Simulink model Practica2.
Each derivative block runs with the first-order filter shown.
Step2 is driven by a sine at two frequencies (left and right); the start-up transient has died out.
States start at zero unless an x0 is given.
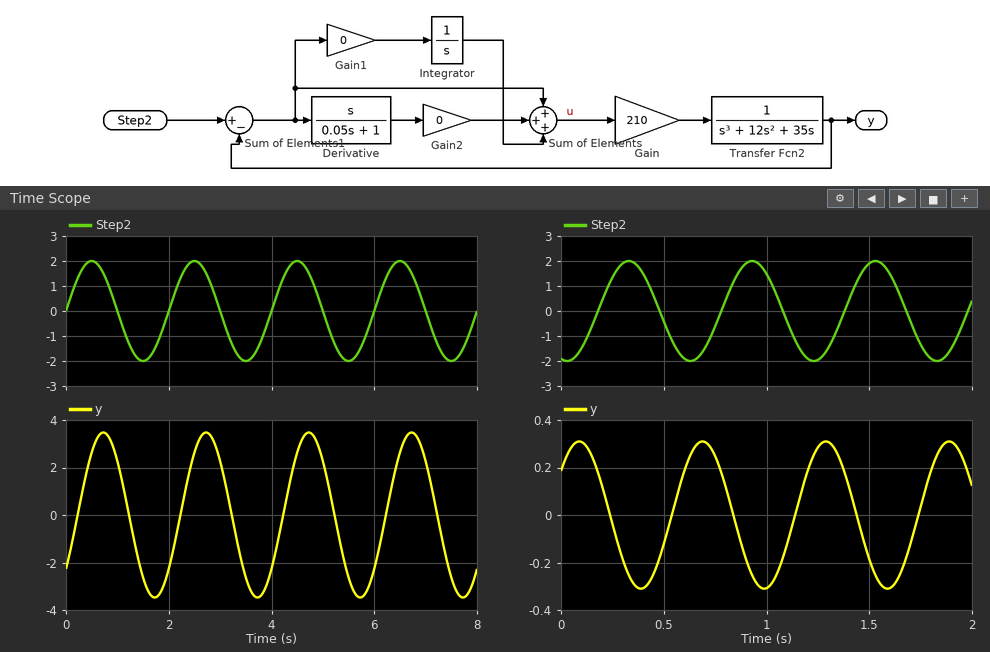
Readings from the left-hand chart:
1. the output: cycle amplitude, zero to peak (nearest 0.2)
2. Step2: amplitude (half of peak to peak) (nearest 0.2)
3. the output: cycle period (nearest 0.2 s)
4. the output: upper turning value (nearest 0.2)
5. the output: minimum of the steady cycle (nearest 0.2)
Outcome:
3.4
2.0
2.0 s
3.4
-3.4
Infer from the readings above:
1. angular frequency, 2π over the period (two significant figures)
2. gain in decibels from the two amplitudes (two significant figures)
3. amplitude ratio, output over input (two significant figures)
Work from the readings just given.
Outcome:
3.1 rad/s
4.6 dB
1.7
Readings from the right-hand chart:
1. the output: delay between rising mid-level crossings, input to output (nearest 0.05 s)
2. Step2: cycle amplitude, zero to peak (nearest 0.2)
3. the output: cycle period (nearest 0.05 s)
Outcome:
0.35 s
2.0
0.60 s
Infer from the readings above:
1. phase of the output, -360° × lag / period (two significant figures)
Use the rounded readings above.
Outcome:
-210°
